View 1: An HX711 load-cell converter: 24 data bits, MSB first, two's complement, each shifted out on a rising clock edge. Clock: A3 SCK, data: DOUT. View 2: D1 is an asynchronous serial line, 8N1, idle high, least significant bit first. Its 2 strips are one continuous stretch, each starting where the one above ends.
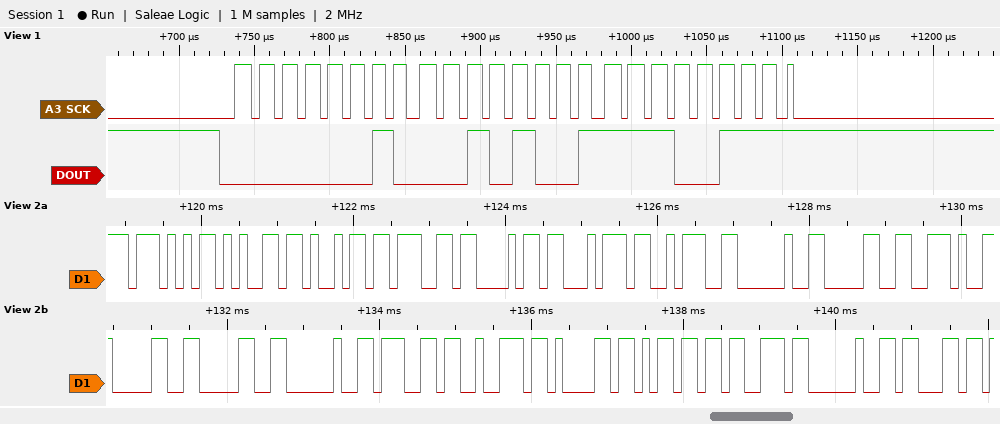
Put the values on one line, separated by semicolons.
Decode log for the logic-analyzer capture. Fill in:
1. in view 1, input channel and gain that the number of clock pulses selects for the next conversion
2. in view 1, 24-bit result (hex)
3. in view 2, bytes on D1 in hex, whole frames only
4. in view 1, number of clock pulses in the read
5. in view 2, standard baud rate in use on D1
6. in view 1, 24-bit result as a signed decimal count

channel A, gain 128; 0x0229E7; 57 65 69 67 68 74 3A 20 30 2E 30 30 20 67 72 61 6D 73 20 63; 25; 9600 baud; 141799
